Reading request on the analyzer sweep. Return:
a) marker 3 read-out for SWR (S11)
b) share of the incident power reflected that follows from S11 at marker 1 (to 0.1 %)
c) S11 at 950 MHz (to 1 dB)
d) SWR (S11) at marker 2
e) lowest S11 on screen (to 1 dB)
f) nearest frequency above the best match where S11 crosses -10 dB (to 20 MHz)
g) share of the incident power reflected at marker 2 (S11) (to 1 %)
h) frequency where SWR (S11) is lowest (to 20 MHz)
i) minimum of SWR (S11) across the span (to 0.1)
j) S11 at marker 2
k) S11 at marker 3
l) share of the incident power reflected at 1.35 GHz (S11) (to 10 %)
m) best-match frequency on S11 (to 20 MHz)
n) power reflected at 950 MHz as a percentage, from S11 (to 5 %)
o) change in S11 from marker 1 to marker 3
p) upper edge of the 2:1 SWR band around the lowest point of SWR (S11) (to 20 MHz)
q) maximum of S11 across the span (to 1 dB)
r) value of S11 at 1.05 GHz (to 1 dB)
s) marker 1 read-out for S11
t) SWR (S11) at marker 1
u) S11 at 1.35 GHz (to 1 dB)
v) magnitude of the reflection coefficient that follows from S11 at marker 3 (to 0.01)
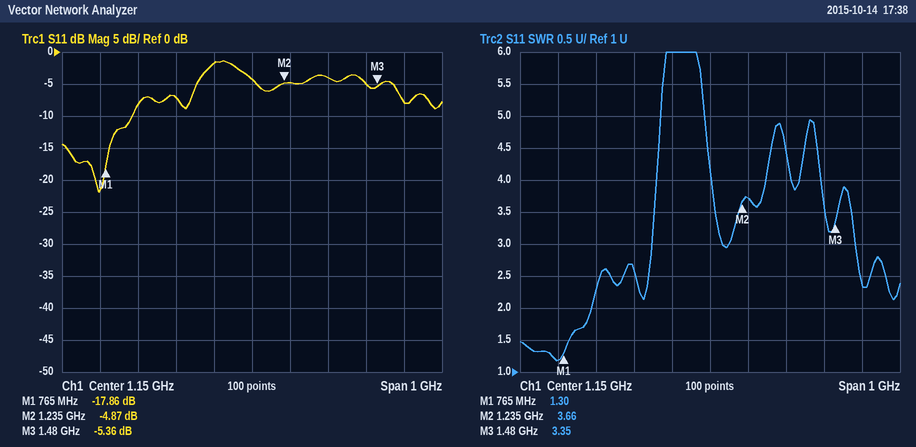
3.35
1.6 %
-7 dB
3.66
-22 dB
840 MHz
33 %
740 MHz
1.2
-4.87 dB
-5.36 dB
40 %
740 MHz
20 %
12.50 dB
840 MHz
-1 dB
-2 dB
-17.86 dB
1.30
-4 dB
0.54
